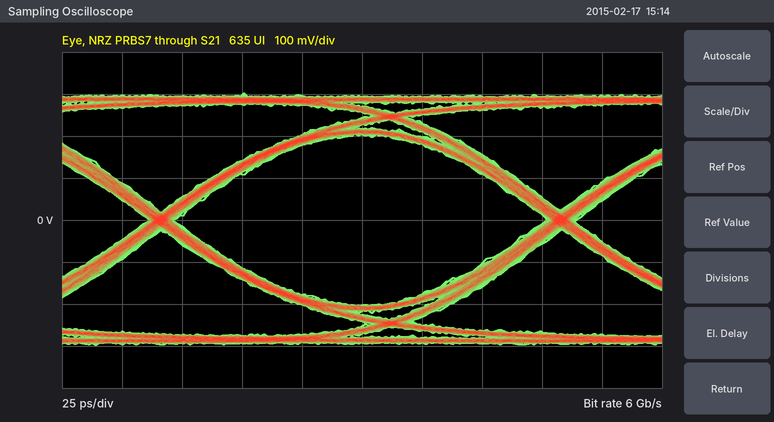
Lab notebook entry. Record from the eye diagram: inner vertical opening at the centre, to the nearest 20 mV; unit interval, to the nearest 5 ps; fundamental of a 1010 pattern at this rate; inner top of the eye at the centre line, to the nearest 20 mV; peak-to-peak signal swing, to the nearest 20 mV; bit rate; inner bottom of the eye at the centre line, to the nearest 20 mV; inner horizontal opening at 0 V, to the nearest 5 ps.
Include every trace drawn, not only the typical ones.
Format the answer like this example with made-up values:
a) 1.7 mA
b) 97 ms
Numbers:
a) 400 mV
b) 165 ps
c) 3 GHz
d) 200 mV
e) 600 mV
f) 6 Gb/s
g) -200 mV
h) 155 ps
